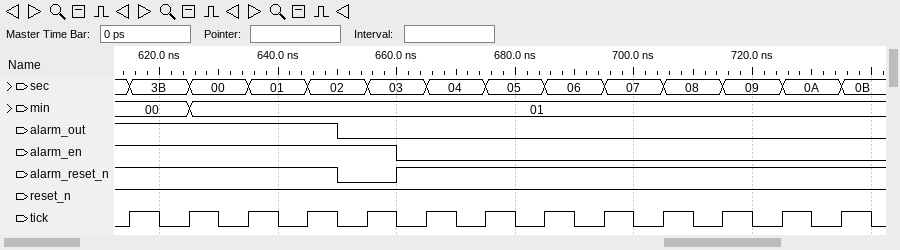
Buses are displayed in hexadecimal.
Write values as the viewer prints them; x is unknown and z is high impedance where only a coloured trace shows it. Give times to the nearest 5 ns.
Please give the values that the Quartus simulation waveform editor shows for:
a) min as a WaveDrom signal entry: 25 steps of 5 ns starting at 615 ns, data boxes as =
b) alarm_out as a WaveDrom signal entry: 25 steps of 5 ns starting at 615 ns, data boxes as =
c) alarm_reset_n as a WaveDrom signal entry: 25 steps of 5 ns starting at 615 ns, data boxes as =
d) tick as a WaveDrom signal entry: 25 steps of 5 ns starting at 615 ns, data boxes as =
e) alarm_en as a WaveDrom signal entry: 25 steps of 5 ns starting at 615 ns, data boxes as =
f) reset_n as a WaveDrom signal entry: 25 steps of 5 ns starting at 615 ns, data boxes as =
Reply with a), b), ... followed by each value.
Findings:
a) {name: 'min', wave: '=.=......................', data: '00 01'}
b) {name: 'alarm_out', wave: '1......0.................'}
c) {name: 'alarm_reset_n', wave: '1......0.1...............'}
d) {name: 'tick', wave: '1010101010101010101010101'}
e) {name: 'alarm_en', wave: '1........0...............'}
f) {name: 'reset_n', wave: '1........................'}
